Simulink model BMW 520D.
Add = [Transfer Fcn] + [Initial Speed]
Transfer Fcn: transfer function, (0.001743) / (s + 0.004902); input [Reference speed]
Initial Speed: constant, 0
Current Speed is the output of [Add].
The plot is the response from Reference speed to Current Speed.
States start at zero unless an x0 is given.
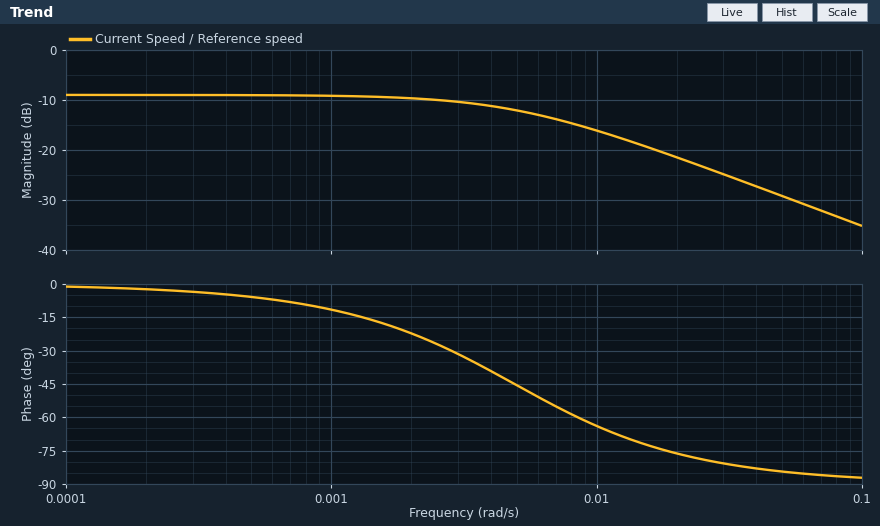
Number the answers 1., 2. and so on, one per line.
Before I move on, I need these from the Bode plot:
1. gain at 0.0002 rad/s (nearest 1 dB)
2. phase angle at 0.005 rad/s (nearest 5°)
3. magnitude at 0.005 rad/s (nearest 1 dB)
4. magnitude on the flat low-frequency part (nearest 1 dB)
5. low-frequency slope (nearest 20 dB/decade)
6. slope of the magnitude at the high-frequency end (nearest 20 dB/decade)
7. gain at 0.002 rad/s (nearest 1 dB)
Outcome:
1. -9 dB
2. -45°
3. -12 dB
4. -9 dB
5. 0 dB/decade
6. -20 dB/decade
7. -10 dB
